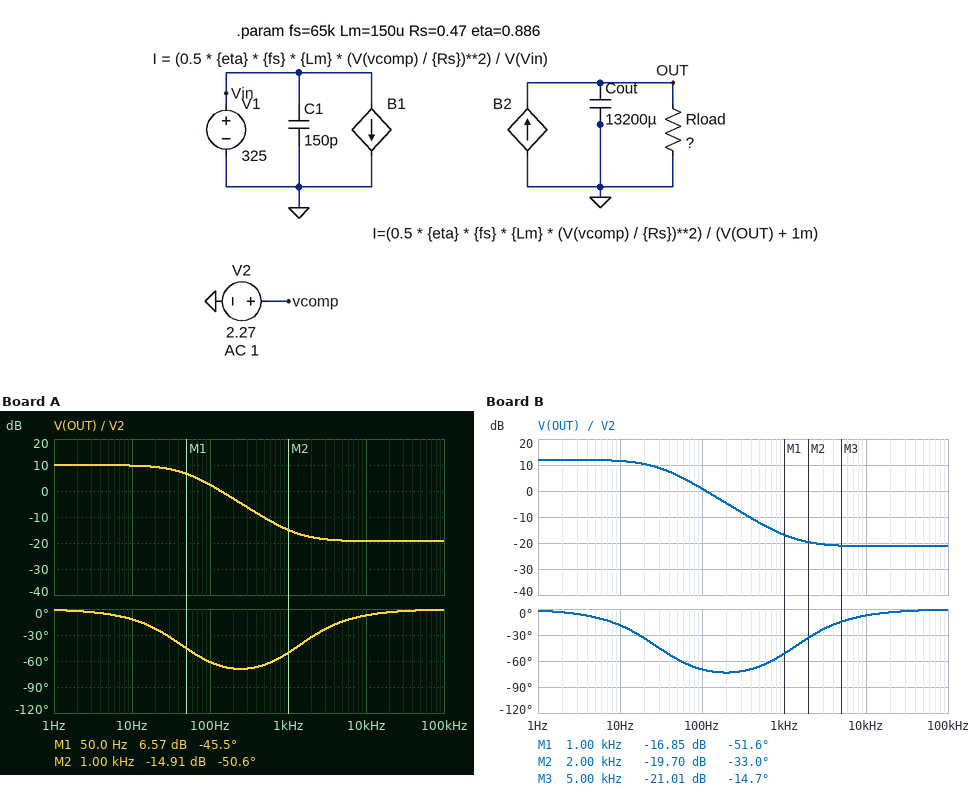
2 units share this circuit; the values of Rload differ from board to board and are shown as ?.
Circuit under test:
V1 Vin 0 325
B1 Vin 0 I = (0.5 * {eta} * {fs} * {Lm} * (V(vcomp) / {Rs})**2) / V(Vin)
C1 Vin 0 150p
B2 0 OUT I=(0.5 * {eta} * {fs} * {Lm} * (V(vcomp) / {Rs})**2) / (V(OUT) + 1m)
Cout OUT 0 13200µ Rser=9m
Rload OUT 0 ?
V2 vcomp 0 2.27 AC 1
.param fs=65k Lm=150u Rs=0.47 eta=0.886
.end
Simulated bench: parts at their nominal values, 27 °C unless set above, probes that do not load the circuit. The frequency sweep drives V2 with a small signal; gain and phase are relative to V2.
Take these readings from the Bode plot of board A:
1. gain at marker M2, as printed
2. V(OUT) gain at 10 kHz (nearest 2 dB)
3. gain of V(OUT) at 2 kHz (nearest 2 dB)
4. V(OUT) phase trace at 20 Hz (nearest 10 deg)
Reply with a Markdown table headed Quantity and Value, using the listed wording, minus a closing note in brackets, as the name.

| Quantity | Value |
|---|---|
| gain at marker M2, as printed | -14.91 dB |
| V(OUT) gain at 10 kHz | -20 dB |
| gain of V(OUT) at 2 kHz | -18 dB |
| V(OUT) phase trace at 20 Hz | -20 deg |
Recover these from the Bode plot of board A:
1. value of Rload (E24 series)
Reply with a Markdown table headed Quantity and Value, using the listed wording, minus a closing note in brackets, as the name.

| Quantity | Value |
|---|---|
| value of Rload | 0.51 Ω |
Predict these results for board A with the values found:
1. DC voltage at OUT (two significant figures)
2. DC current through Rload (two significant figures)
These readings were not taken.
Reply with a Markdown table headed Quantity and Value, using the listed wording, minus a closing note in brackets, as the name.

| Quantity | Value |
|---|---|
| DC voltage at OUT | 7.2 V |
| DC current through Rload | 14 A |
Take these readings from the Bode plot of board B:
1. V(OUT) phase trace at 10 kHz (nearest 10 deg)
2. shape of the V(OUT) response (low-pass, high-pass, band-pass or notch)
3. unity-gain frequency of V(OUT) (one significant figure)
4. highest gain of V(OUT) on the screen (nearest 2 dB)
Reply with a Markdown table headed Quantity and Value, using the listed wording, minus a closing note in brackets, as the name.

| Quantity | Value |
|---|---|
| V(OUT) phase trace at 10 kHz | -10 deg |
| shape of the V(OUT) response | low-pass |
| unity-gain frequency of V(OUT) | 100 Hz |
| highest gain of V(OUT) on the screen | 12 dB |
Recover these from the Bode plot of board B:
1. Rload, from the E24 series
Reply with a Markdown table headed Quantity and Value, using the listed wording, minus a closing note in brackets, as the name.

| Quantity | Value |
|---|---|
| Rload, from the E24 series | 0.82 Ω |
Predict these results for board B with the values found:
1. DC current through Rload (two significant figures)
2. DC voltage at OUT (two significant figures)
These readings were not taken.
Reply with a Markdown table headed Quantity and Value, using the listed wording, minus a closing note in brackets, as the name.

| Quantity | Value |
|---|---|
| DC current through Rload | 11 A |
| DC voltage at OUT | 9.1 V |
